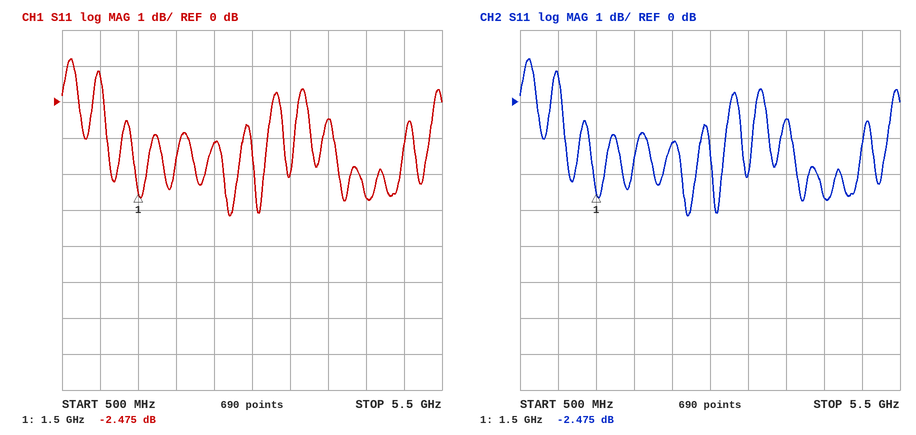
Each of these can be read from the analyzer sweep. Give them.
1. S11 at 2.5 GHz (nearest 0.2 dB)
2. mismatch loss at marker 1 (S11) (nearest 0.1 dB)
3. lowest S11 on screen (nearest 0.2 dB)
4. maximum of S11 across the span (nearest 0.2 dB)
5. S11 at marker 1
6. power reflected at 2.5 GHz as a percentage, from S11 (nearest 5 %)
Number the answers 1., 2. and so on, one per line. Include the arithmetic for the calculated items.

1. -1.2 dB
2. −10 log10(1 − 10^(-2.475/10)) ≈ 3.6 dB
3. -3.2 dB
4. 1.2 dB
5. -2.475 dB
6. 10^(-1.2/10) ≈ 75.9 %, so 75 % to the nearest 5 %
